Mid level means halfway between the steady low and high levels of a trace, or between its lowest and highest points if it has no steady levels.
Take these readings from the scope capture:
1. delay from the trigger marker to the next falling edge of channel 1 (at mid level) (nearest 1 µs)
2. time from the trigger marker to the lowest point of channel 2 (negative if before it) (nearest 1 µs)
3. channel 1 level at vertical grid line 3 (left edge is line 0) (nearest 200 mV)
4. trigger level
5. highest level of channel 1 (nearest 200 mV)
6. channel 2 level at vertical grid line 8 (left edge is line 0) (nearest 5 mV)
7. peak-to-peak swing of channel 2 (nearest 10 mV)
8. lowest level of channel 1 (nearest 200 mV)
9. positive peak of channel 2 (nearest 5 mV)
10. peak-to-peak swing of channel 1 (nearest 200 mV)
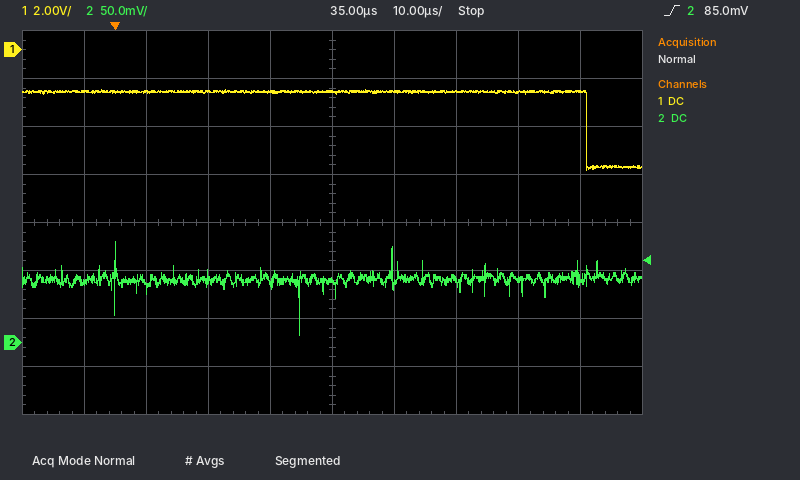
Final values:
76 µs
+30 µs
-1.8 V
85.0 mV
-1.6 V
65 mV
100 mV
-5.0 V
105 mV
3.4 V
